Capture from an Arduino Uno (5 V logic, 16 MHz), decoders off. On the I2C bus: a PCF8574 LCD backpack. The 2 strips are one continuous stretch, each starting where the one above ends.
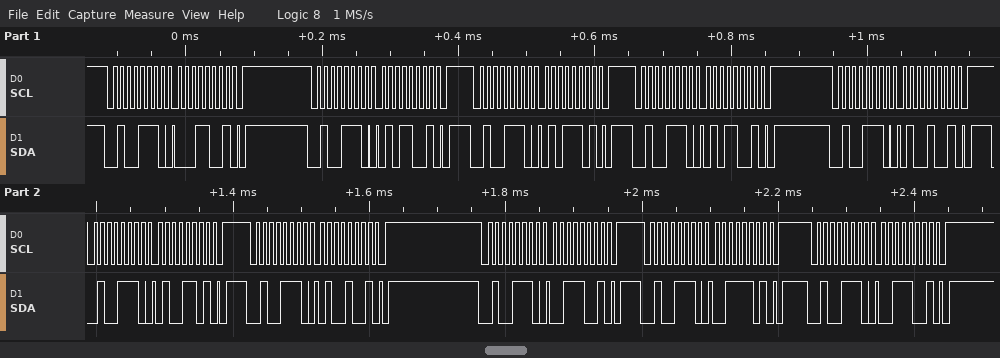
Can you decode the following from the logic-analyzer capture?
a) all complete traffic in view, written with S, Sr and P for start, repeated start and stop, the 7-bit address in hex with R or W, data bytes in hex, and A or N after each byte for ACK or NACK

S 27W A 19 A P S 27W A 59 A P S 27W A 5D A P S 27W A 59 A P S 27W A 49 A P S 27W A 4D A P S 27W A 49 A P S 27W A 39 A P S 27W A 3D A P S 27W A 39 A P
